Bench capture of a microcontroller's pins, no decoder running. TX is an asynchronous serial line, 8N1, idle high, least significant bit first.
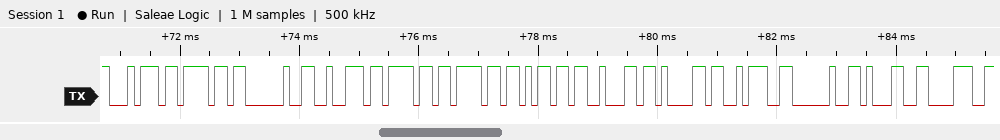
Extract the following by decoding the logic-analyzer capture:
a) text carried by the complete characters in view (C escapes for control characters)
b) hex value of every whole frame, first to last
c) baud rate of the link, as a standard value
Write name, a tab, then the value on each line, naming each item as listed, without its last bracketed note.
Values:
text carried by the complete characters in view	"to roomba: 18"
hex value of every whole frame, first to last	0x74 0x6F 0x20 0x72 0x6F 0x6F 0x6D 0x62 0x61 0x3A 0x20 0x31 0x38
baud rate of the link, as a standard value	9600 baud
